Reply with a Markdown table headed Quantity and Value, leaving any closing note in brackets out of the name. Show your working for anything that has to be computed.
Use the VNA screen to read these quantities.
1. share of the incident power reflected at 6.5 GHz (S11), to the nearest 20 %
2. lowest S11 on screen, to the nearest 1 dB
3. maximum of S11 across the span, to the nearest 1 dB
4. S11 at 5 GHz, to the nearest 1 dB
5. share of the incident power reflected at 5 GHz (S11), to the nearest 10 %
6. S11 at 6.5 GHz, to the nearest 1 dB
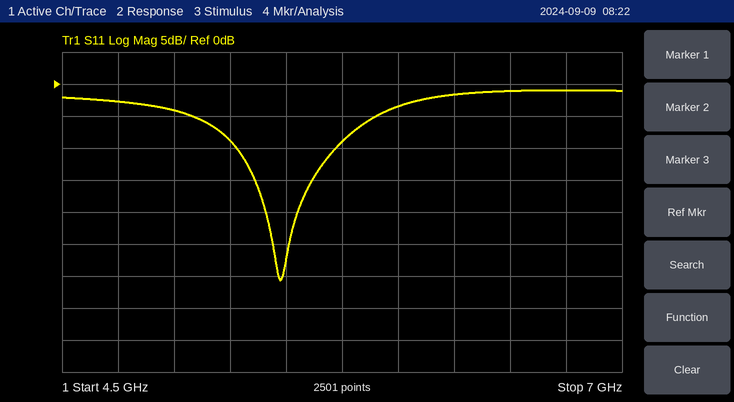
| Quantity | Value |
|---|---|
| share of the incident power reflected at 6.5 GHz (S11), to the nearest 20 % | 10^(-1/10) ≈ 79.4 %, so 80 % to the nearest 20 % |
| lowest S11 on screen, to the nearest 1 dB | -31 dB |
| maximum of S11 across the span, to the nearest 1 dB | -1 dB |
| S11 at 5 GHz, to the nearest 1 dB | -4 dB |
| share of the incident power reflected at 5 GHz (S11), to the nearest 10 % | 10^(-4/10) ≈ 40 % |
| S11 at 6.5 GHz, to the nearest 1 dB | -1 dB |
